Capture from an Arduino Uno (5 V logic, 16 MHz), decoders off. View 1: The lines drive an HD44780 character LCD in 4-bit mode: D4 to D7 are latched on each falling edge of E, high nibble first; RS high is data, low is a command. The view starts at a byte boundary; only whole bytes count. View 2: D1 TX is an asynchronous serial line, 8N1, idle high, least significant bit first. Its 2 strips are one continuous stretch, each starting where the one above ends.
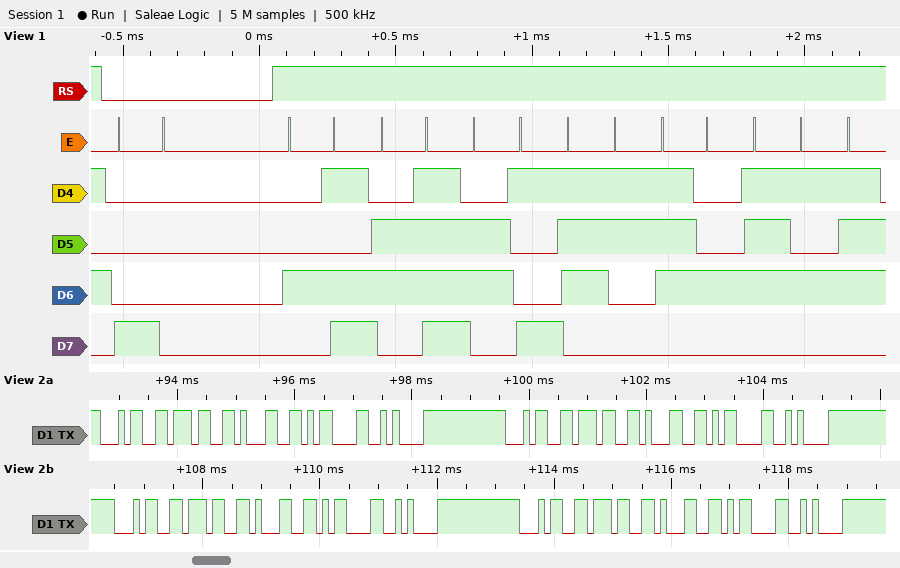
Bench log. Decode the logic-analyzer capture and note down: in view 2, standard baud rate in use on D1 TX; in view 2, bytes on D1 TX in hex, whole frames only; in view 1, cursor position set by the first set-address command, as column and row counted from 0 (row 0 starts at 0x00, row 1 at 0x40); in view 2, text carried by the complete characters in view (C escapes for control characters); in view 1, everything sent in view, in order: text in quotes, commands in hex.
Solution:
9600 baud
34 37 31 0D 0A 34 37 31 0D 0A 34 37 31 0D 0A 34 37 31 0D 0A
column 0, row 0
"471\r\n471\r\n471\r\n471\r\n"
0x80 "Moistu"
